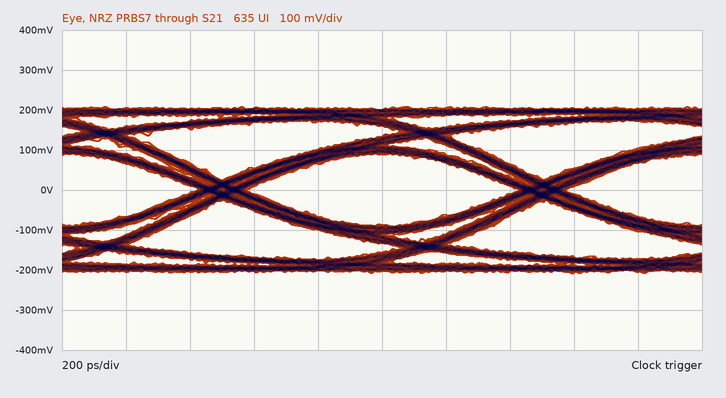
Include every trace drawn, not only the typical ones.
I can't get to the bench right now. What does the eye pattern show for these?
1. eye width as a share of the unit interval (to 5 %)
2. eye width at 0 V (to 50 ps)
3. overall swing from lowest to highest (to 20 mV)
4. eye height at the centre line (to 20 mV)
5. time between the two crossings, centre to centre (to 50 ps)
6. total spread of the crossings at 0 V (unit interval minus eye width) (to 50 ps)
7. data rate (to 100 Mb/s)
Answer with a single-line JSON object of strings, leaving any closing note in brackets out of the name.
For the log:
{"eye width as a share of the unit interval": "85 %", "eye width at 0 V": "850 ps", "overall swing from lowest to highest": "420 mV", "eye height at the centre line": "180 mV", "time between the two crossings, centre to centre": "1.00 ns", "total spread of the crossings at 0 V (unit interval minus eye width)": "150 ps", "data rate": "1.0 Gb/s"}
